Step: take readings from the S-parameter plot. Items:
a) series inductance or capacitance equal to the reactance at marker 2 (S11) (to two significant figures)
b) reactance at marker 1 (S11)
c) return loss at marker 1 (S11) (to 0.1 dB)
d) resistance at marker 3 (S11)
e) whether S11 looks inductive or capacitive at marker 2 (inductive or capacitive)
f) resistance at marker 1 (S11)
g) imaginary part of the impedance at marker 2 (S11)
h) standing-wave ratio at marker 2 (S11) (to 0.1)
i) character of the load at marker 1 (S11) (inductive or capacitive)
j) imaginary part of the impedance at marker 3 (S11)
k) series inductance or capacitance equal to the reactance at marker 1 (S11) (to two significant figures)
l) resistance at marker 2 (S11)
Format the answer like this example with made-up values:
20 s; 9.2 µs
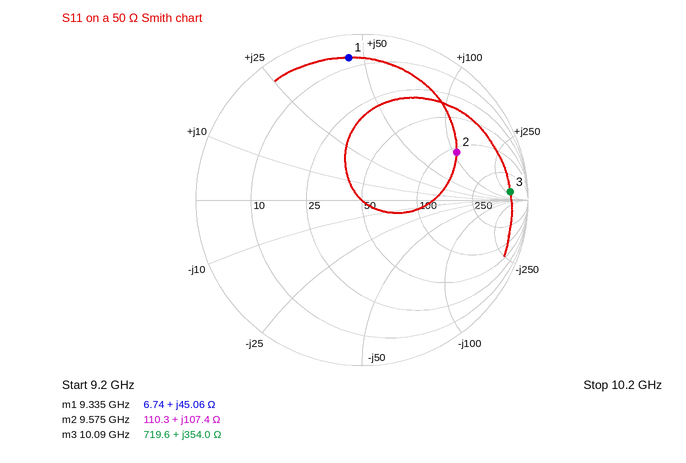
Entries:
1.8 nH; +45.06 Ω; 1.3 dB; 719.6 Ω; inductive; 6.74 Ω; +107.4 Ω; 4.5; inductive; +354.0 Ω; 770 pH; 110.3 Ω
